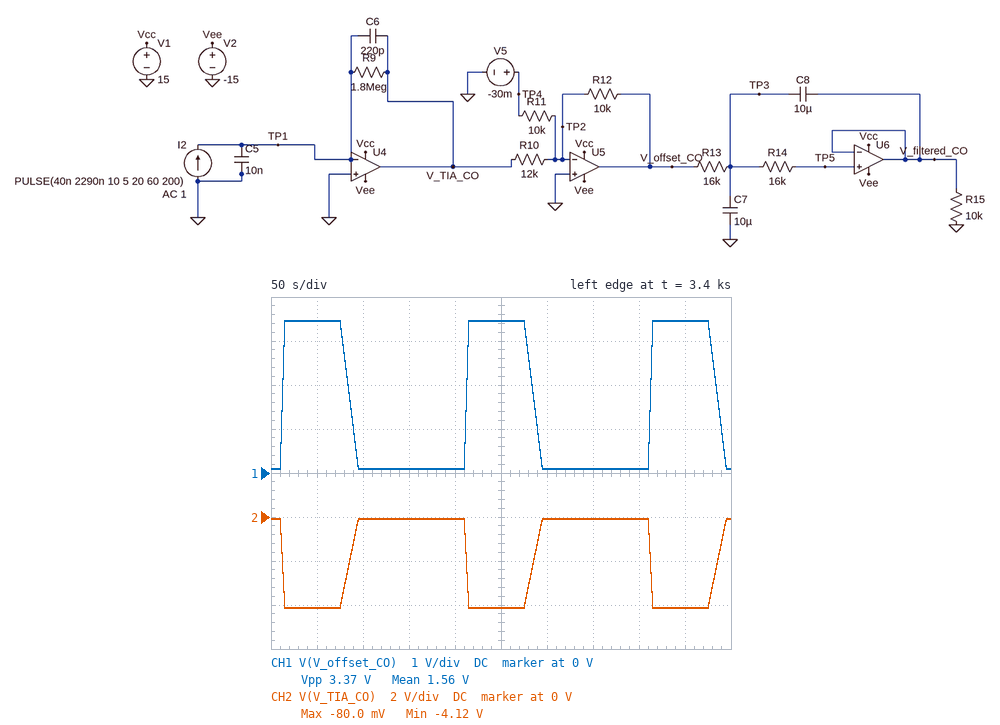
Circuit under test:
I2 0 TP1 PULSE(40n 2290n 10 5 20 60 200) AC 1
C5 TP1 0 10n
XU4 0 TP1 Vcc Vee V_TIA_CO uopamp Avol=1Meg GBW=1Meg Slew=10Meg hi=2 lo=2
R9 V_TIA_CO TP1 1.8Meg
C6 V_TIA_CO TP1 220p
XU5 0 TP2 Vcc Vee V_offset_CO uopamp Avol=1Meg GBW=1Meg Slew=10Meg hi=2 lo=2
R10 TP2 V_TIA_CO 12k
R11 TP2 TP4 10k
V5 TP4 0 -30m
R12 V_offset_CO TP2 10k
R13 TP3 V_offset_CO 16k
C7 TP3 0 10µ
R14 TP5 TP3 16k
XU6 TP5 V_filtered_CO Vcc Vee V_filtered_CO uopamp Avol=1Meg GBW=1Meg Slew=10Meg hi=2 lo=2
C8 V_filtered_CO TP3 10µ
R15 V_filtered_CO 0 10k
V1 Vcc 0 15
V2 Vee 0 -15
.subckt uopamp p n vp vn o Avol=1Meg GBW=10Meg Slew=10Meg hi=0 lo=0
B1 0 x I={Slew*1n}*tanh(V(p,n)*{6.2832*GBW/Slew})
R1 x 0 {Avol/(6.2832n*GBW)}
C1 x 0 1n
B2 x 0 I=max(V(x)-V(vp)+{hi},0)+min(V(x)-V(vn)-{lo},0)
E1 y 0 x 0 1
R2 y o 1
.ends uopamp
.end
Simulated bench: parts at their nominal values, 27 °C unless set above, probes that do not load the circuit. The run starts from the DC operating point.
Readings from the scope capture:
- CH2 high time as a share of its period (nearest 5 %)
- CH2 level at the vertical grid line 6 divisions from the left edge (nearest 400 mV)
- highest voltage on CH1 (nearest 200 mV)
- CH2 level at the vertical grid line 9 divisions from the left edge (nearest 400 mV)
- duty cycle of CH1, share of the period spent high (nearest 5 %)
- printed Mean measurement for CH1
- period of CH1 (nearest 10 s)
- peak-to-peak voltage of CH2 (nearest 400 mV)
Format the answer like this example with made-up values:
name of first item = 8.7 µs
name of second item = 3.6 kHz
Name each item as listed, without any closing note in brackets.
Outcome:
CH2 high time as a share of its period = 65 %
CH2 level at the vertical grid line 6 divisions from the left edge = 0 V
highest voltage on CH1 = 3.4 V
CH2 level at the vertical grid line 9 divisions from the left edge = -4.0 V
duty cycle of CH1, share of the period spent high = 35 %
printed Mean measurement for CH1 = 1.56 V
period of CH1 = 200 s
peak-to-peak voltage of CH2 = 4.0 V
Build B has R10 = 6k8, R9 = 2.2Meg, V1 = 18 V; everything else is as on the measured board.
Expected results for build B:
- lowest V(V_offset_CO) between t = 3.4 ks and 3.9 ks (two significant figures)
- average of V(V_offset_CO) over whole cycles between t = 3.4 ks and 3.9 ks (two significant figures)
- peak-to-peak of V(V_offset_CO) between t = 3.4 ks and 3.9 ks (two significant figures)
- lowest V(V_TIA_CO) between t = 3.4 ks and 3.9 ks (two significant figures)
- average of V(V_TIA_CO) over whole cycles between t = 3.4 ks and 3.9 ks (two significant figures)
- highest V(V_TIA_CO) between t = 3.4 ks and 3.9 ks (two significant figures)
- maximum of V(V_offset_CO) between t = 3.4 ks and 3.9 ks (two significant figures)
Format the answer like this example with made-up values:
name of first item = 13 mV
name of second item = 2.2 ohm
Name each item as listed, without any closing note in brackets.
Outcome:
lowest V(V_offset_CO) between t = 3.4 ks and 3.9 ks = 160 mV
average of V(V_offset_CO) over whole cycles between t = 3.4 ks and 3.9 ks = 2.8 V
peak-to-peak of V(V_offset_CO) between t = 3.4 ks and 3.9 ks = 7.3 V
lowest V(V_TIA_CO) between t = 3.4 ks and 3.9 ks = -5.0 V
average of V(V_TIA_CO) over whole cycles between t = 3.4 ks and 3.9 ks = -1.9 V
highest V(V_TIA_CO) between t = 3.4 ks and 3.9 ks = -88 mV
maximum of V(V_offset_CO) between t = 3.4 ks and 3.9 ks = 7.4 V
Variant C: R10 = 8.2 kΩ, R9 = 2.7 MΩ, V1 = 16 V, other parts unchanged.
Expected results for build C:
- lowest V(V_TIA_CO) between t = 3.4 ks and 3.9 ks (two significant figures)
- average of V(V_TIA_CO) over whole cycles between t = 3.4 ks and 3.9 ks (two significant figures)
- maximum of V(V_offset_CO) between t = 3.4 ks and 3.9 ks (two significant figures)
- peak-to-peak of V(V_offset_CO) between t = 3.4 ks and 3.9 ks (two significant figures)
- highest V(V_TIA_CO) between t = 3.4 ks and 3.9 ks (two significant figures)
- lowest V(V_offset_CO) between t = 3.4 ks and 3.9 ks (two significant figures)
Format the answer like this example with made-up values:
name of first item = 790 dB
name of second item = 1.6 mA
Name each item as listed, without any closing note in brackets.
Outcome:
lowest V(V_TIA_CO) between t = 3.4 ks and 3.9 ks = -6.2 V
average of V(V_TIA_CO) over whole cycles between t = 3.4 ks and 3.9 ks = -2.3 V
maximum of V(V_offset_CO) between t = 3.4 ks and 3.9 ks = 7.6 V
peak-to-peak of V(V_offset_CO) between t = 3.4 ks and 3.9 ks = 7.4 V
highest V(V_TIA_CO) between t = 3.4 ks and 3.9 ks = -110 mV
lowest V(V_offset_CO) between t = 3.4 ks and 3.9 ks = 160 mV
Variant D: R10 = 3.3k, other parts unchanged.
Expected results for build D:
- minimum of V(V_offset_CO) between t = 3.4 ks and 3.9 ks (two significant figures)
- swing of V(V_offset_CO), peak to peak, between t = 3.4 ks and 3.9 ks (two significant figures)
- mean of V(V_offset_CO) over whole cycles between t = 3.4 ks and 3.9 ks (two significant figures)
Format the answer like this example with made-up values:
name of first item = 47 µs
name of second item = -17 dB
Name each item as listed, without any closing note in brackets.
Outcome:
minimum of V(V_offset_CO) between t = 3.4 ks and 3.9 ks = 250 mV
swing of V(V_offset_CO), peak to peak, between t = 3.4 ks and 3.9 ks = 12 V
mean of V(V_offset_CO) over whole cycles between t = 3.4 ks and 3.9 ks = 4.7 V
